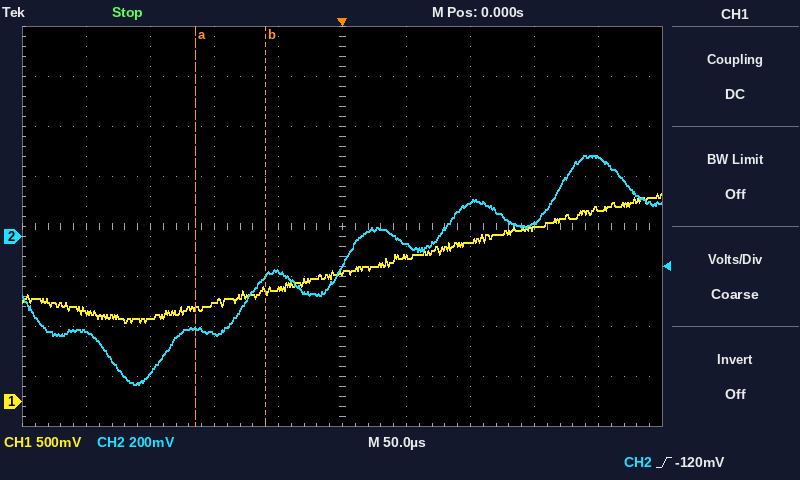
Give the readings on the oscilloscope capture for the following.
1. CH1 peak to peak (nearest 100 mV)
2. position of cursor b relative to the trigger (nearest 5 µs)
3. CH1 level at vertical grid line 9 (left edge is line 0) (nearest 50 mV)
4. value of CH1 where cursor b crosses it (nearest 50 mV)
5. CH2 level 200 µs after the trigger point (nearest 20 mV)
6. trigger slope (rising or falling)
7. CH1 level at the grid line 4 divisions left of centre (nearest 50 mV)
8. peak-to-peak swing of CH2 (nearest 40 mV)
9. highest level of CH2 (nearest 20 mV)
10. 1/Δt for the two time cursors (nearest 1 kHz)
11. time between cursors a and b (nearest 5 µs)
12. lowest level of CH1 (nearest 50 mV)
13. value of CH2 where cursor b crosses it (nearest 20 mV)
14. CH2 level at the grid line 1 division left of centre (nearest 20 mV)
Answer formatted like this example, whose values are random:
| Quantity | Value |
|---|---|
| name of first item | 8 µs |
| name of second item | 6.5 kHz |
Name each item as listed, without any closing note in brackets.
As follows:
| Quantity | Value |
|---|---|
| CH1 peak to peak | 1.30 V |
| position of cursor b relative to the trigger | -60 µs |
| CH1 level at vertical grid line 9 (left edge is line 0) | 1.95 V |
| value of CH1 where cursor b crosses it | 1.10 V |
| CH2 level 200 µs after the trigger point | 320 mV |
| trigger slope | rising |
| CH1 level at the grid line 4 divisions left of centre | 900 mV |
| peak-to-peak swing of CH2 | 920 mV |
| highest level of CH2 | 320 mV |
| 1/Δt for the two time cursors | 18 kHz |
| time between cursors a and b | 55 µs |
| lowest level of CH1 | 800 mV |
| value of CH2 where cursor b crosses it | -160 mV |
| CH2 level at the grid line 1 division left of centre | -140 mV |
